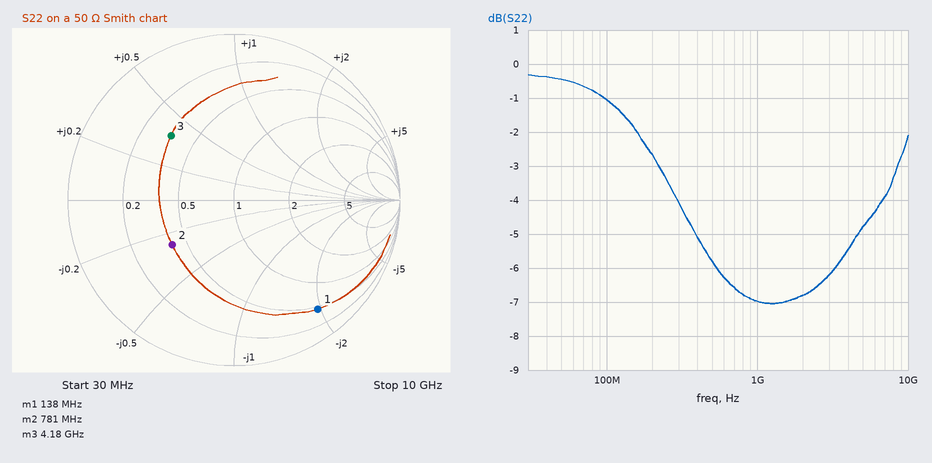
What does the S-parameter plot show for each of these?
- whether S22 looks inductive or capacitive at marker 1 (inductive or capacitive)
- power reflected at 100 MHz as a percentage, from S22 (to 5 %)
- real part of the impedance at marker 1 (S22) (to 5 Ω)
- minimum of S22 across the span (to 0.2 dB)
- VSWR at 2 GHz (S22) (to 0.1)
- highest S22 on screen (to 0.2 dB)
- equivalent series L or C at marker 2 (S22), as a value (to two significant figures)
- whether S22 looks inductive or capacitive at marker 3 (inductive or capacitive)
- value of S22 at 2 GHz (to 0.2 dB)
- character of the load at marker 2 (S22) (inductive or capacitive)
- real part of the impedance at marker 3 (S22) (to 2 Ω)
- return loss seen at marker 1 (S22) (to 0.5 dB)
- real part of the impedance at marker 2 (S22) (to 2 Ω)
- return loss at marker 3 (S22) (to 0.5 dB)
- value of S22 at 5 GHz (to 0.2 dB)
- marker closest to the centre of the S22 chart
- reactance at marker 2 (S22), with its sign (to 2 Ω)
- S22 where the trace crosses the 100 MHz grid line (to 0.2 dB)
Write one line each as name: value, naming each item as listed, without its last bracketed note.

whether S22 looks inductive or capacitive at marker 1: capacitive
power reflected at 100 MHz as a percentage, from S22: 80 %
real part of the impedance at marker 1 (S22): 25 Ω
minimum of S22 across the span: -7.0 dB
VSWR at 2 GHz (S22): 2.7
highest S22 on screen: -0.4 dB
equivalent series L or C at marker 2 (S22), as a value: 15 pF
whether S22 looks inductive or capacitive at marker 3: inductive
value of S22 at 2 GHz: -6.8 dB
character of the load at marker 2 (S22): capacitive
real part of the impedance at marker 3 (S22): 18 Ω
return loss seen at marker 1 (S22): 1.5 dB
real part of the impedance at marker 2 (S22): 20 Ω
return loss at marker 3 (S22): 5.5 dB
value of S22 at 5 GHz: -4.8 dB
marker closest to the centre of the S22 chart: marker 2
reactance at marker 2 (S22), with its sign: -14 Ω
S22 where the trace crosses the 100 MHz grid line: -1.0 dB
